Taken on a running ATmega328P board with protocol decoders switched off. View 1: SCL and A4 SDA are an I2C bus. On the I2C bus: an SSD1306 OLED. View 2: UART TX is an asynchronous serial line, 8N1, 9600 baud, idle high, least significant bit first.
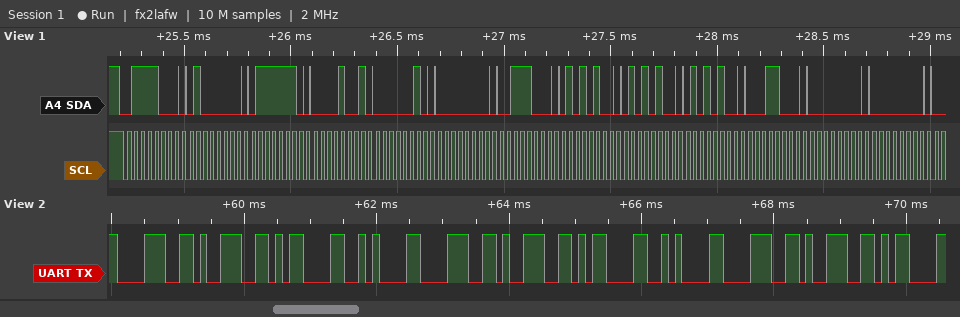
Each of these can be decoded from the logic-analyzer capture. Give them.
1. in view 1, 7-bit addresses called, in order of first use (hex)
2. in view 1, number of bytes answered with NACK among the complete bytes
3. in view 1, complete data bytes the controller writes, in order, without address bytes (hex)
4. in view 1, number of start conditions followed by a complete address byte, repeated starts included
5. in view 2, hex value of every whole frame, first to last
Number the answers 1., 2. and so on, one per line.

1. 0x3C
2. 0
3. 40 7E 09 02 00 38 54 54 54 18 00 00
4. 1
5. 38 39 0D 0A 38 39 0D 0A 38 39 0D
